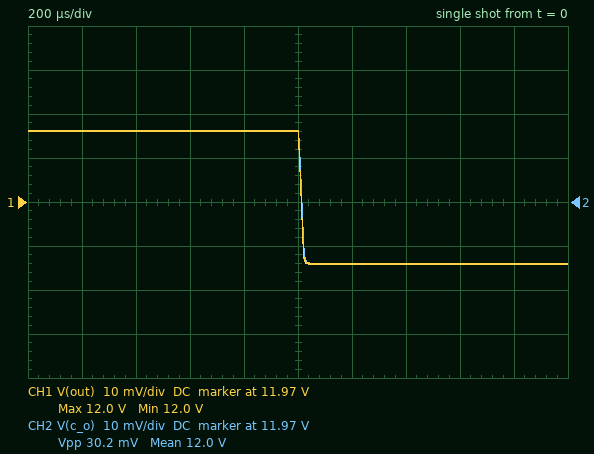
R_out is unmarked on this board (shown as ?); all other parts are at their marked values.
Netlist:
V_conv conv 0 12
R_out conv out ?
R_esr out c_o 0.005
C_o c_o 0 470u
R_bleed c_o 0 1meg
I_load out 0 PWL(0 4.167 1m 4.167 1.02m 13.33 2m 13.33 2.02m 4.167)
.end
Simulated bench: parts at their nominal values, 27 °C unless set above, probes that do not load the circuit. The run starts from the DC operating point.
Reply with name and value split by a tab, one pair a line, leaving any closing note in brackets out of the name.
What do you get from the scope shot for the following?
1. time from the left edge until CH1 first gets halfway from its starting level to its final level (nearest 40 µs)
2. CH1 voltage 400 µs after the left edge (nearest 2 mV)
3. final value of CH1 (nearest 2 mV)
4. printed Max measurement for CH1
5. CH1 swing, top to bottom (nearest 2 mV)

time from the left edge until CH1 first gets halfway from its starting level to its final level	1.00 ms
CH1 voltage 400 µs after the left edge	11.986 V
final value of CH1	11.956 V
printed Max measurement for CH1	12.0 V
CH1 swing, top to bottom	30 mV
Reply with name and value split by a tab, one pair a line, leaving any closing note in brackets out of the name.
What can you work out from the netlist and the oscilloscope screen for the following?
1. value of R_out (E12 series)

value of R_out	3.3 mΩ
